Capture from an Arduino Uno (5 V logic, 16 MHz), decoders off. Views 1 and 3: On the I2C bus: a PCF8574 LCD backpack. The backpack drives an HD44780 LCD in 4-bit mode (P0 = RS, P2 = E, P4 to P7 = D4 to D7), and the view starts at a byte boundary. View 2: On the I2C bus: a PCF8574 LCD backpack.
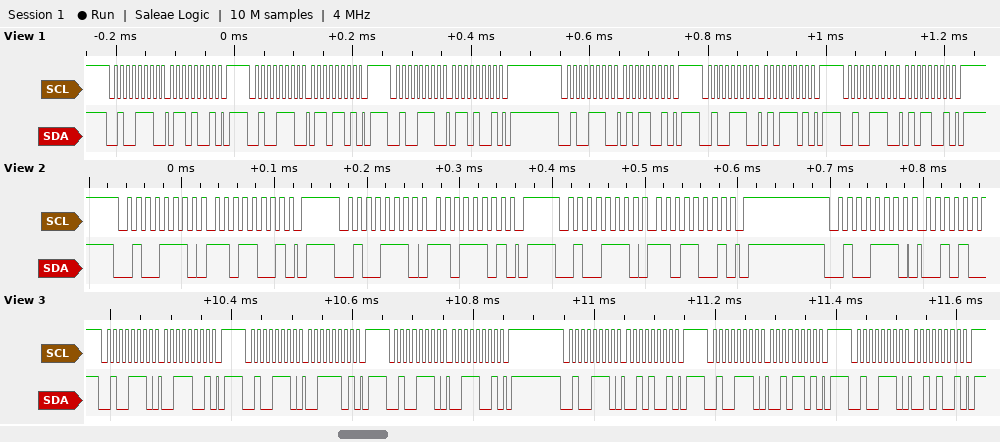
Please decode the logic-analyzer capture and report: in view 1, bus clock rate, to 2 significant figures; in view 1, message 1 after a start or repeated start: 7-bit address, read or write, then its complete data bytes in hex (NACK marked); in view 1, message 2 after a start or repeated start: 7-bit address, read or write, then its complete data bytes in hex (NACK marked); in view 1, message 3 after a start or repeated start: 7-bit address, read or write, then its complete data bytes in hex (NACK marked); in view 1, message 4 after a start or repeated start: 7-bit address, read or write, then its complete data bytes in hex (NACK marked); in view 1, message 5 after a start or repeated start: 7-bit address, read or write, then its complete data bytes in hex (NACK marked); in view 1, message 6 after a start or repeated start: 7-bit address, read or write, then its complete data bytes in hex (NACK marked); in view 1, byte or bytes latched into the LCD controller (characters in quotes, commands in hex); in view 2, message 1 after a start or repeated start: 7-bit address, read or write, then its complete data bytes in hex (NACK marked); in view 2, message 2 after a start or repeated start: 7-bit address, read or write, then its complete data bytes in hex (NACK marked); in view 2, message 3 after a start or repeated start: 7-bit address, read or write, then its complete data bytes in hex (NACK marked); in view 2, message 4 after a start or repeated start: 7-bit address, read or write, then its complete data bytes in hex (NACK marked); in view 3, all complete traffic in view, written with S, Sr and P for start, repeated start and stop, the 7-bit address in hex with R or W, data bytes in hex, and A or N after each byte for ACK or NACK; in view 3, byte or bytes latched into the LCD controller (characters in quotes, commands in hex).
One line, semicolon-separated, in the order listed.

100 kHz; 0x27 write: 69; 0x27 write: 6D; 0x27 write: 69; 0x27 write: 59; 0x27 write: 5D; 0x27 write: 59; 'e'; 0x27 write: D9; 0x27 write: DD; 0x27 write: D9; 0x27 write; S 27W A 39 A P S 27W A 3D A P S 27W A 39 A P S 27W A 29 A P S 27W A 2D A P S 27W A 29 A P; '2'
